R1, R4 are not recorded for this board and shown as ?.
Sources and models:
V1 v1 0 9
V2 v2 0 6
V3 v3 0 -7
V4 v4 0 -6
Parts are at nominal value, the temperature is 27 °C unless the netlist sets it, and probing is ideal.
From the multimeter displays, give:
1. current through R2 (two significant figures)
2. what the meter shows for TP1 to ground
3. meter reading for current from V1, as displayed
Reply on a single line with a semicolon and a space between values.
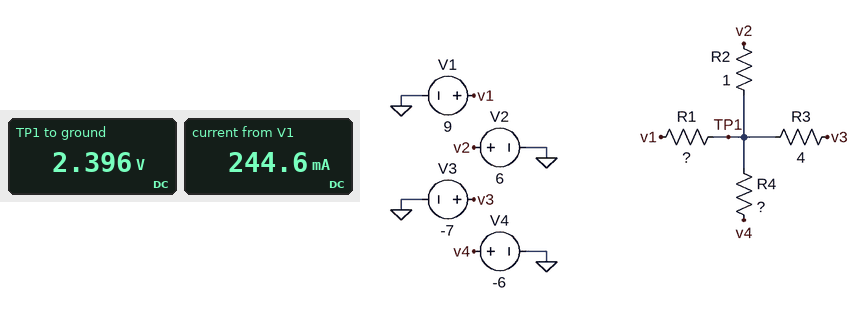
3.6 A; 2.396 V; 244.6 mA
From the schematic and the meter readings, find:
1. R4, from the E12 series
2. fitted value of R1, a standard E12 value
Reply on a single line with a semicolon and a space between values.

5.6 Ω; 27 Ω
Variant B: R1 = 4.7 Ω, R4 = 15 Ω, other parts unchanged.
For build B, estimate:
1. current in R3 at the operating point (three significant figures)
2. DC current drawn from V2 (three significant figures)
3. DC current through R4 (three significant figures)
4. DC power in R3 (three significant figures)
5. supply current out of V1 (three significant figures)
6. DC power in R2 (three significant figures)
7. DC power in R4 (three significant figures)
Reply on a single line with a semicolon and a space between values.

2.69 A; 2.23 A; 651 mA; 29.0 W; 1.11 A; 4.98 W; 6.36 W
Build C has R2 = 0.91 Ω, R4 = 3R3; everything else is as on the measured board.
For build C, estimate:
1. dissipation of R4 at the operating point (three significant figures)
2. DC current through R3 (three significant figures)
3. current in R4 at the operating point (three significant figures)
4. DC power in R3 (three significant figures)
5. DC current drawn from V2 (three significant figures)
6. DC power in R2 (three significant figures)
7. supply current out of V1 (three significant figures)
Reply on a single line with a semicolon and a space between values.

19.3 W; 2.25 A; 2.42 A; 20.2 W; 4.41 A; 17.7 W; 260 mA
